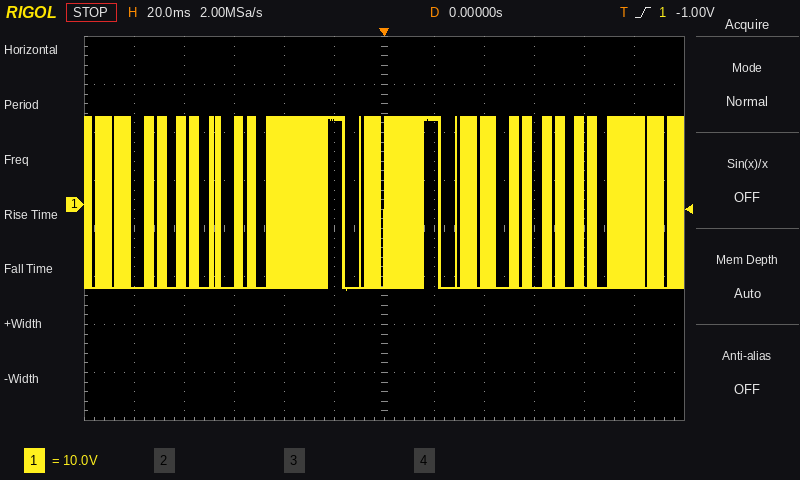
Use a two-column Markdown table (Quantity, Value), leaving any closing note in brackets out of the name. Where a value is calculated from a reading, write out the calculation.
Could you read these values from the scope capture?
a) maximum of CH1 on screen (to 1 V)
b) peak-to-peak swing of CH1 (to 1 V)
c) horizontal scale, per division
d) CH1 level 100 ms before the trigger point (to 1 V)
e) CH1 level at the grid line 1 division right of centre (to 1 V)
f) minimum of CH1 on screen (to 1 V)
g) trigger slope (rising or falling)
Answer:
| Quantity | Value |
|---|---|
| maximum of CH1 on screen | 18 V |
| peak-to-peak swing of CH1 | 18 V − (-18 V) = 36 V |
| horizontal scale, per division | 20 ms |
| CH1 level 100 ms before the trigger point | -17 V |
| CH1 level at the grid line 1 division right of centre | 18 V |
| minimum of CH1 on screen | -18 V |
| trigger slope | rising |
